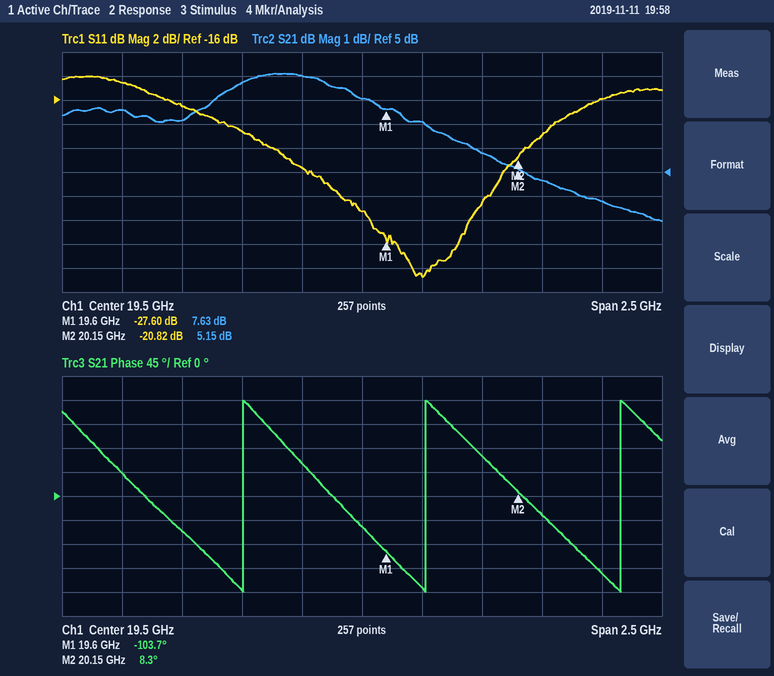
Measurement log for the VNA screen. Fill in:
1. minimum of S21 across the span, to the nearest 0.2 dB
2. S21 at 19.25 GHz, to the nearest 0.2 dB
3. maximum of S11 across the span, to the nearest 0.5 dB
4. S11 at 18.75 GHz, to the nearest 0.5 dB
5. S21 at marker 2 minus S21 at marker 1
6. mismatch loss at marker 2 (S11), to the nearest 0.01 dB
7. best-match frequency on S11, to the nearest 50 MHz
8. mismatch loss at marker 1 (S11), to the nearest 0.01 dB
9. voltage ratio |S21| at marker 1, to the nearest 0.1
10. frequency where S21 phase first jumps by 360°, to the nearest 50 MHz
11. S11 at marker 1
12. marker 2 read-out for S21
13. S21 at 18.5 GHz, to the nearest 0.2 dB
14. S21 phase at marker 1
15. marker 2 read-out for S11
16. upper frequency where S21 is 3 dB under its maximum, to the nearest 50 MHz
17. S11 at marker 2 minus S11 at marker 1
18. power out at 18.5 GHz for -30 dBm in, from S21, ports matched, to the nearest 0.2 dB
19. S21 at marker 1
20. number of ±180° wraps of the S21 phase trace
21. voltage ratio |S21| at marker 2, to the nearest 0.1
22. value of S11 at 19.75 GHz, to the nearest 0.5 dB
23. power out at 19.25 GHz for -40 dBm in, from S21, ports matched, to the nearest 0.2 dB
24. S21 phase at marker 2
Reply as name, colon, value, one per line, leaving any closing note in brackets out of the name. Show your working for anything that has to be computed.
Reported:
minimum of S21 across the span, to the nearest 0.2 dB: 3.0 dB
S21 at 19.25 GHz, to the nearest 0.2 dB: 9.0 dB
maximum of S11 across the span, to the nearest 0.5 dB: -14.0 dB
S11 at 18.75 GHz, to the nearest 0.5 dB: -16.5 dB
S21 at marker 2 minus S21 at marker 1: 5.15 − (7.63) = -2.48 dB
mismatch loss at marker 2 (S11), to the nearest 0.01 dB: −10 log10(1 − 10^(-20.82/10)) ≈ 0.04 dB
best-match frequency on S11, to the nearest 50 MHz: 19.75 GHz
mismatch loss at marker 1 (S11), to the nearest 0.01 dB: −10 log10(1 − 10^(-27.6/10)) ≈ 0.01 dB
voltage ratio |S21| at marker 1, to the nearest 0.1: 10^(7.63/20) ≈ 2.4
frequency where S21 phase first jumps by 360°, to the nearest 50 MHz: 19.00 GHz
S11 at marker 1: -27.60 dB
marker 2 read-out for S21: 5.15 dB
S21 at 18.5 GHz, to the nearest 0.2 dB: 7.6 dB
S21 phase at marker 1: -103.7°
marker 2 read-out for S11: -20.82 dB
upper frequency where S21 is 3 dB under its maximum, to the nearest 50 MHz: 19.95 GHz
S11 at marker 2 minus S11 at marker 1: -20.82 − (-27.6) = 6.78 dB
power out at 18.5 GHz for -30 dBm in, from S21, ports matched, to the nearest 0.2 dB: -30 dBm + (7.6 dB) = -22.4 dBm
S21 at marker 1: 7.63 dB
number of ±180° wraps of the S21 phase trace: 3
voltage ratio |S21| at marker 2, to the nearest 0.1: 10^(5.15/20) ≈ 1.8
value of S11 at 19.75 GHz, to the nearest 0.5 dB: -30.5 dB
power out at 19.25 GHz for -40 dBm in, from S21, ports matched, to the nearest 0.2 dB: -40 dBm + (9.0 dB) = -31.0 dBm
S21 phase at marker 2: 8.3°
